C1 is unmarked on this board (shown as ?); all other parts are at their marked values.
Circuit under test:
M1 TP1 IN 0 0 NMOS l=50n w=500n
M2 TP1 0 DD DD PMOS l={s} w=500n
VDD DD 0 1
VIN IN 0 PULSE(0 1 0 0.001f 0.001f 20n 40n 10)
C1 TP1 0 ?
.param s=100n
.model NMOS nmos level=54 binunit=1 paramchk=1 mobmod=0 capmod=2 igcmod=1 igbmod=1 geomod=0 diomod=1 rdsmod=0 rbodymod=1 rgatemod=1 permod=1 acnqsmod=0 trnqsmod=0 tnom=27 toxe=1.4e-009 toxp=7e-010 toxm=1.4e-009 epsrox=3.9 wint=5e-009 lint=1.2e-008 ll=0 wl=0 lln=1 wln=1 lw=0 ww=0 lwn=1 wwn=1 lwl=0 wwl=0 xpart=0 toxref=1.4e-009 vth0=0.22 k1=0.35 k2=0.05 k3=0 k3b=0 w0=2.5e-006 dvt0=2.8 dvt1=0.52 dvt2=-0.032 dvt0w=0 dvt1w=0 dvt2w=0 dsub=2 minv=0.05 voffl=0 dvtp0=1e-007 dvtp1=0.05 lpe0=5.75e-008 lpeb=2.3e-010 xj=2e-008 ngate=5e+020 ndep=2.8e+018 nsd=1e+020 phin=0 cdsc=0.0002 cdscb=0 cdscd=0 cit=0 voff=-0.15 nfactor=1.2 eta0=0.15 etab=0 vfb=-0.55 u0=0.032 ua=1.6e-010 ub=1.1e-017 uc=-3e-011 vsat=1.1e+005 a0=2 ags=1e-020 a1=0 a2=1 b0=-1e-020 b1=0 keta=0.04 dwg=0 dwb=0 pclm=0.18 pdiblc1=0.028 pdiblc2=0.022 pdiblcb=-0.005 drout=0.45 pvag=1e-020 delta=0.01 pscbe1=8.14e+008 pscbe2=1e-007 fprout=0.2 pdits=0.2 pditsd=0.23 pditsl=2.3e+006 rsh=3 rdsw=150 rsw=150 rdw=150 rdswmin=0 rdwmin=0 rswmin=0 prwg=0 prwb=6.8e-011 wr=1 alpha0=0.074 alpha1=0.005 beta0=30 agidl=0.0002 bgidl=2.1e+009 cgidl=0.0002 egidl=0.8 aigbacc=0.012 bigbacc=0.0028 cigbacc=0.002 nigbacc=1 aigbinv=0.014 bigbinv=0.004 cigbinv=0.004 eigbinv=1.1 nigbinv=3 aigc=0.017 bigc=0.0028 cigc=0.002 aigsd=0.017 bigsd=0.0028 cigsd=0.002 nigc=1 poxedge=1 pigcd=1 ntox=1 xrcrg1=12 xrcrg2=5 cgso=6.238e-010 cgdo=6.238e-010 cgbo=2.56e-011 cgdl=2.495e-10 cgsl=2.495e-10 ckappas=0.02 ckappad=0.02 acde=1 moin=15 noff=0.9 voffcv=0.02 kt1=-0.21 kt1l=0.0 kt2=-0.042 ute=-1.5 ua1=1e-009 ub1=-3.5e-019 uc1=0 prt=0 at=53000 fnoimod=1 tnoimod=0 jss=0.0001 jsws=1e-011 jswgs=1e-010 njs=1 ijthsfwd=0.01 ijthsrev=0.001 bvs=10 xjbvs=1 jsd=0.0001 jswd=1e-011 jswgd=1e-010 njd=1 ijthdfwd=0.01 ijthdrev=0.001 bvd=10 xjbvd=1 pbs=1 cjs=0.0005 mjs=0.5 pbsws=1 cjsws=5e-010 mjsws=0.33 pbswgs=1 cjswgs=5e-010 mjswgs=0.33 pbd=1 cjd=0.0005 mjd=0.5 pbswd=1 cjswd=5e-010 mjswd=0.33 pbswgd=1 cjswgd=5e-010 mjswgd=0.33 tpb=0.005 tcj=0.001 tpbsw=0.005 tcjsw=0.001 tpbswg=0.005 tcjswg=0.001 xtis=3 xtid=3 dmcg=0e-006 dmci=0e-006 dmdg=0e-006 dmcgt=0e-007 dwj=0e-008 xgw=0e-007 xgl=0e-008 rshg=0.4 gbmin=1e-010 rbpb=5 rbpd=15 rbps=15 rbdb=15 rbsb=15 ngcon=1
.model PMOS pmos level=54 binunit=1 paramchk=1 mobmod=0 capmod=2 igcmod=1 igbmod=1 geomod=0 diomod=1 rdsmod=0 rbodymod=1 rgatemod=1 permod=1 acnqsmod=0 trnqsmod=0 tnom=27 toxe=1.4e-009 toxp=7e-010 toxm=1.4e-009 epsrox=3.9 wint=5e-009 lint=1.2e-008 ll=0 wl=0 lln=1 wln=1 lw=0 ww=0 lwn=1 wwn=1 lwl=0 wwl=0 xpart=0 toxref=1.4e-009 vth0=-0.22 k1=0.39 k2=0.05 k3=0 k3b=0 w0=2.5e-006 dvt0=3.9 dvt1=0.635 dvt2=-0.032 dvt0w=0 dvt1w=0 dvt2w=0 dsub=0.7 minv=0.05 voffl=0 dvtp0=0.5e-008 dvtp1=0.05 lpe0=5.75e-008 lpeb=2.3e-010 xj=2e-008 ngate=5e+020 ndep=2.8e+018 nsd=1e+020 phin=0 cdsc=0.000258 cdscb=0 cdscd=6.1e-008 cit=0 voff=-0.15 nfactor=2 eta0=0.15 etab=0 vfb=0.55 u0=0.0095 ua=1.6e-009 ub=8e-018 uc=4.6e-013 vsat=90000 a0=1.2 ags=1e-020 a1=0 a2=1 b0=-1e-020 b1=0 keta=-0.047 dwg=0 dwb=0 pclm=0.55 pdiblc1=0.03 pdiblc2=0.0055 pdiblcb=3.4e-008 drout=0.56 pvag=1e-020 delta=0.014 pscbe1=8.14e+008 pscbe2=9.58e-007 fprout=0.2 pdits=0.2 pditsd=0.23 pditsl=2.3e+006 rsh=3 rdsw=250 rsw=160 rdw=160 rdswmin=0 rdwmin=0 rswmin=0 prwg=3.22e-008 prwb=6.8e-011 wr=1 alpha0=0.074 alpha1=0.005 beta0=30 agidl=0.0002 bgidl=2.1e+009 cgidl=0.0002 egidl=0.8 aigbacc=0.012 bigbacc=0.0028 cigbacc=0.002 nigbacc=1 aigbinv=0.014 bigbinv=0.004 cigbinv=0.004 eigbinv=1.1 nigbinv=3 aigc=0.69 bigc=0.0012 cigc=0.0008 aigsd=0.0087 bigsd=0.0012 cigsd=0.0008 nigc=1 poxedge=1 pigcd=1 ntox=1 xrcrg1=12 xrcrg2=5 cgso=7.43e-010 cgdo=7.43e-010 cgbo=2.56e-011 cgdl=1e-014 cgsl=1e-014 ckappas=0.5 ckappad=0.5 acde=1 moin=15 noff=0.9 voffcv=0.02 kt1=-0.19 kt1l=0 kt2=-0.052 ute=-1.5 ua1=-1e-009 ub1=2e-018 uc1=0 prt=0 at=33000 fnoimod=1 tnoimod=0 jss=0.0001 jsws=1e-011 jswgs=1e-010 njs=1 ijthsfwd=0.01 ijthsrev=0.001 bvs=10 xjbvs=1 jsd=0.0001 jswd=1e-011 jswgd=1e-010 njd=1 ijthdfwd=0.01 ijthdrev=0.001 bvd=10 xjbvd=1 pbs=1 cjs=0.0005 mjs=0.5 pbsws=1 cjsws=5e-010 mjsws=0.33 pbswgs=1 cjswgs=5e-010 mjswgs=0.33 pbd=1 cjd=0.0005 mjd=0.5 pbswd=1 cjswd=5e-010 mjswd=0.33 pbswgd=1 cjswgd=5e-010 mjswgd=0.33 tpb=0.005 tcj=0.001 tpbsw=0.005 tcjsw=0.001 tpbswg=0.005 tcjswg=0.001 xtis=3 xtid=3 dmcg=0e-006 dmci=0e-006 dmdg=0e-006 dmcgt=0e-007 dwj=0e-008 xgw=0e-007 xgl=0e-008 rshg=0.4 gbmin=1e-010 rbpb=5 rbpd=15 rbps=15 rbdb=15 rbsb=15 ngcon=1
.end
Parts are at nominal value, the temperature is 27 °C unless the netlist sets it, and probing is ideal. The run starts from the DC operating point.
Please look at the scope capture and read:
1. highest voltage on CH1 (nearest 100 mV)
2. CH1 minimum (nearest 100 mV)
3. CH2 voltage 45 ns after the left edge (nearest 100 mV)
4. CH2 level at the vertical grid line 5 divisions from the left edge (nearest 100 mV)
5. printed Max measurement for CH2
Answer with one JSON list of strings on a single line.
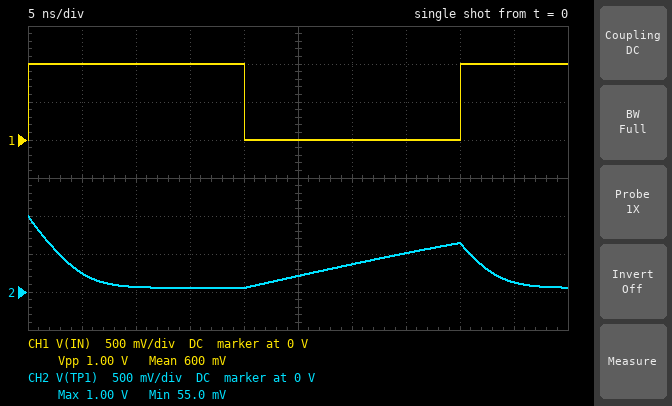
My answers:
["1.0 V", "0 V", "100 mV", "200 mV", "1.00 V"]
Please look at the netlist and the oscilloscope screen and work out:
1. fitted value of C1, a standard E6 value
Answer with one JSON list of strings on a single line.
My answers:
["1.5 pF"]
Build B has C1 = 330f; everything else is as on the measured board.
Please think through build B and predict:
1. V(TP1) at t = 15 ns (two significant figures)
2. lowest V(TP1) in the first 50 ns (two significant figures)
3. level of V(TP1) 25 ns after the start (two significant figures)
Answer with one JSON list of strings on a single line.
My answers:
["53 mV", "51 mV", "700 mV"]
